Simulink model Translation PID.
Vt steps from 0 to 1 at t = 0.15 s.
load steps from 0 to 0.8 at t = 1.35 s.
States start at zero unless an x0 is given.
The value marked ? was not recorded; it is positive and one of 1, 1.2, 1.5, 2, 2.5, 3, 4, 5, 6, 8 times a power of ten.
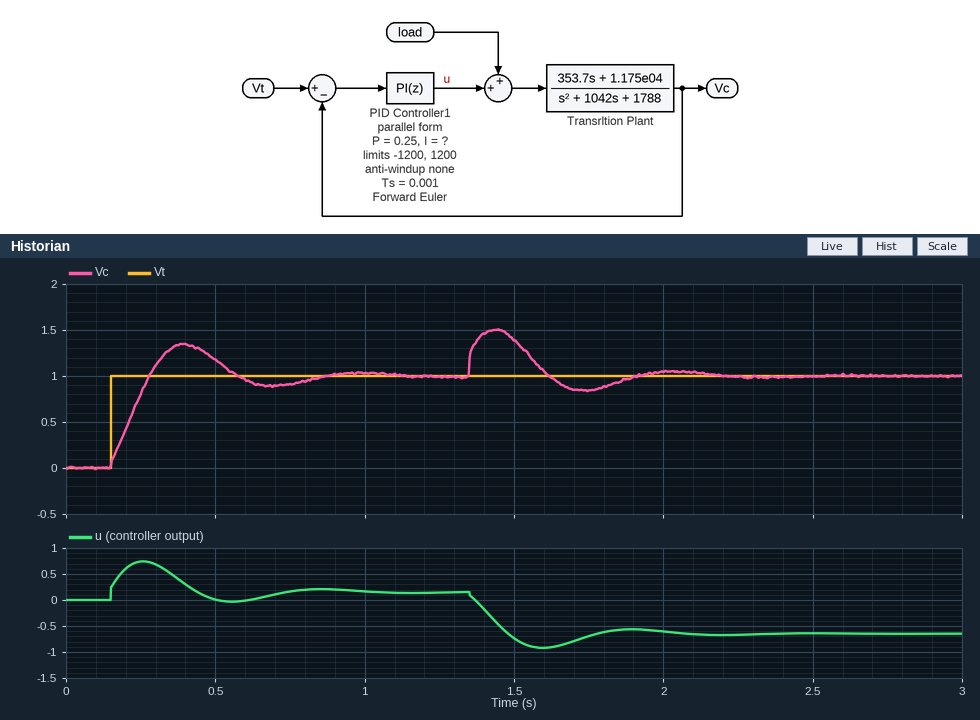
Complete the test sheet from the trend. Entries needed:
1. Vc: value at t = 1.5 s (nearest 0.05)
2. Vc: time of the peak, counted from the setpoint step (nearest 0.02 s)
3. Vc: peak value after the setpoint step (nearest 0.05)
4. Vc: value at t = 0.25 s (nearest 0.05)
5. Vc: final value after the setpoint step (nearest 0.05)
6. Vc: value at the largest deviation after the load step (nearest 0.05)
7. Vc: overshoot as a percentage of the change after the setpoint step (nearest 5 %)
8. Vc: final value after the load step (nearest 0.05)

1.40
0.24 s
1.35
0.80
1.00
1.50
35 %
1.00
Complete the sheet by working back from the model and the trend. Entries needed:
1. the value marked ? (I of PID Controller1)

12
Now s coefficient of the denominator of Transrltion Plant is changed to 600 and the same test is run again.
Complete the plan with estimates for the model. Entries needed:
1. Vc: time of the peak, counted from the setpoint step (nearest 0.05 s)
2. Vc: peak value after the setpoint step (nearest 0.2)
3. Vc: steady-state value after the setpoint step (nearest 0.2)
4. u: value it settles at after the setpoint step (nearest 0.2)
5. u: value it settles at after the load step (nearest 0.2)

0.20 s
1.2
1.0
0.2
-0.6
